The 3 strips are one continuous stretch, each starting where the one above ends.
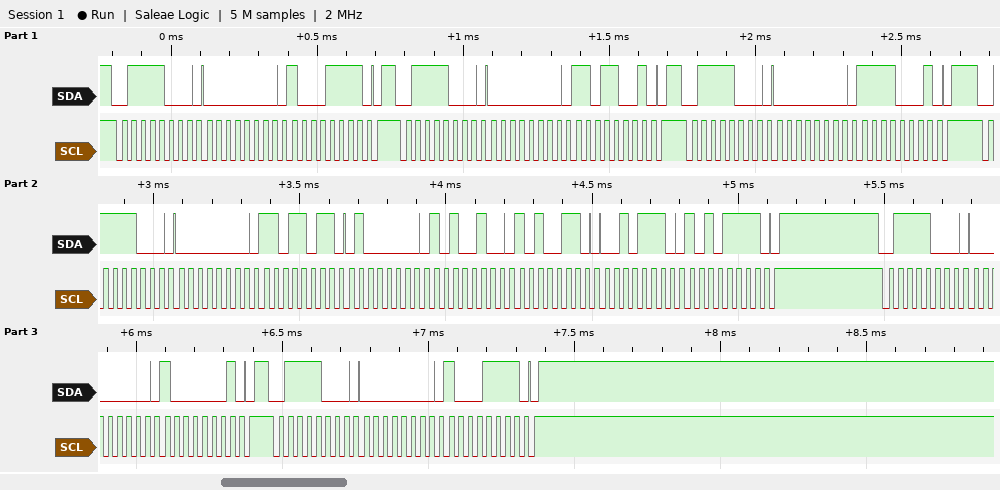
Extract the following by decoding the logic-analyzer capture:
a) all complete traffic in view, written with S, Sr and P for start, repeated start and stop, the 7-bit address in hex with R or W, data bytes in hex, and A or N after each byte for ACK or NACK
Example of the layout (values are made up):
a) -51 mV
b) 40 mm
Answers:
a) S 3CW A 00 A 8F A P S 3CW A 00 A D9 A P S 3CW A 00 A F1 A P S 3CW A 00 A DB A 40 A A4 A A6 A 2E A AF A P S 3CW A 00 A 81 A P S 3CW A 00 A 8F A P
